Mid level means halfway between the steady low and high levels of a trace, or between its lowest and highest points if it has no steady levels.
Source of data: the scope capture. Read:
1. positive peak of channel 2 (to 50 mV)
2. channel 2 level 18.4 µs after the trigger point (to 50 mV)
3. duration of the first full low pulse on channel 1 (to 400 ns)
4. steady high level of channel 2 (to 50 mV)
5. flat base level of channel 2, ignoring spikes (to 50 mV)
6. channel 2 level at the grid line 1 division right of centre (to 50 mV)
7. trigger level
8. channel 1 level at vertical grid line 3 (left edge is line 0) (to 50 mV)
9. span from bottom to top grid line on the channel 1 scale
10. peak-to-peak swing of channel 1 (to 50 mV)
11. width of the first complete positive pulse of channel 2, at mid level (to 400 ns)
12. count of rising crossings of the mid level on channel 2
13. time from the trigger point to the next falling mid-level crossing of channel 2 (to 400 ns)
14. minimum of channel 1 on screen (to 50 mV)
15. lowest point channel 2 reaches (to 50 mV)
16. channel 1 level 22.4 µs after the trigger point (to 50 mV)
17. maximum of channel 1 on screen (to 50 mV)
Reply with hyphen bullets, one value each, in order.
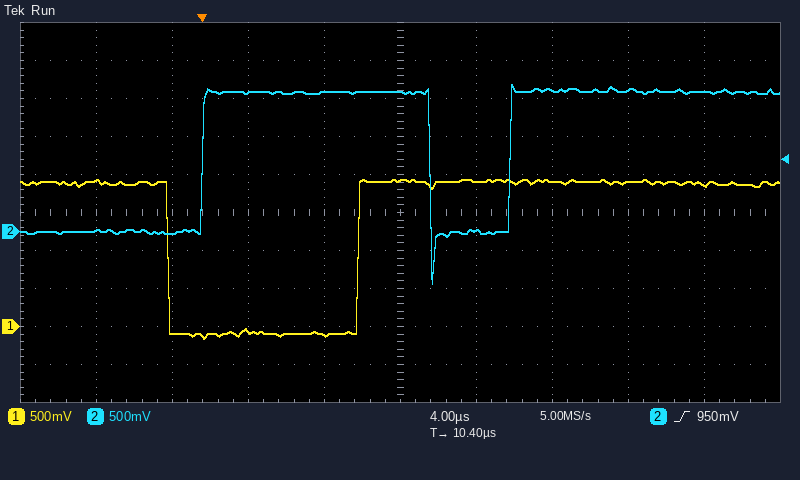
- 1.95 V
- 1.85 V
- 10.0 µs
- 1.85 V
- 0 mV
- 0 mV
- 950 mV
- -50 mV
- 5 V
- 2.10 V
- 12.0 µs
- 2
- 12.0 µs
- -150 mV
- -700 mV
- 1.90 V
- 1.95 V
